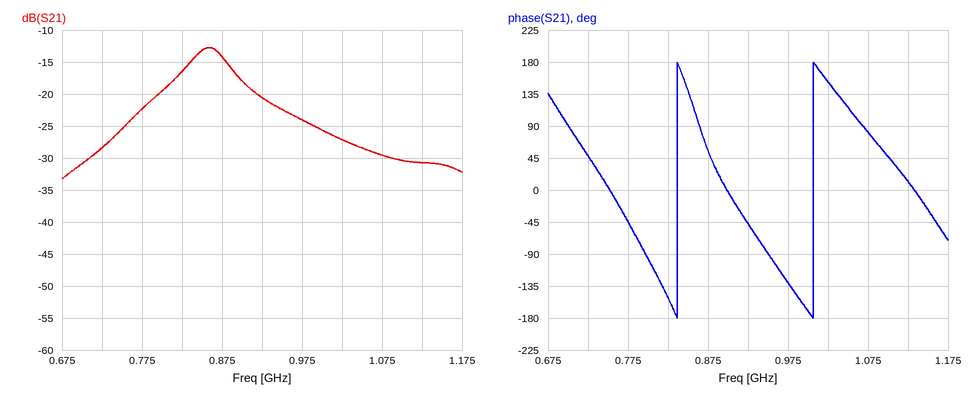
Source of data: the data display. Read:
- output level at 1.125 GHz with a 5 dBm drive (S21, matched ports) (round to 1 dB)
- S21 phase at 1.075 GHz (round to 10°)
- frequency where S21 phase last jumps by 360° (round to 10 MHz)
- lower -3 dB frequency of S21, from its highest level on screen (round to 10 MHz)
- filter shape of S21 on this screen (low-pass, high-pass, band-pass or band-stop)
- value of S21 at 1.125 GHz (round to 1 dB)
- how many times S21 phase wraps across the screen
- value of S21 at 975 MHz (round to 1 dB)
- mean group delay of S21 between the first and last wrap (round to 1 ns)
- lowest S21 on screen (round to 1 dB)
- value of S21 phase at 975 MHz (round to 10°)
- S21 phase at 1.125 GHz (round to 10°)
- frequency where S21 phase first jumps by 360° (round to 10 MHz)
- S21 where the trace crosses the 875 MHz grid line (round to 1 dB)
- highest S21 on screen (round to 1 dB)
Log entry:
-26 dBm
80°
1.01 GHz
830 MHz
band-pass
-31 dB
2
-24 dB
6 ns
-33 dB
-130°
10°
840 MHz
-14 dB
-13 dB
